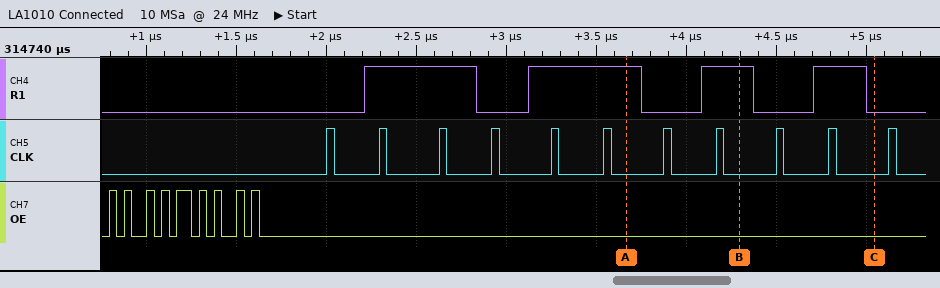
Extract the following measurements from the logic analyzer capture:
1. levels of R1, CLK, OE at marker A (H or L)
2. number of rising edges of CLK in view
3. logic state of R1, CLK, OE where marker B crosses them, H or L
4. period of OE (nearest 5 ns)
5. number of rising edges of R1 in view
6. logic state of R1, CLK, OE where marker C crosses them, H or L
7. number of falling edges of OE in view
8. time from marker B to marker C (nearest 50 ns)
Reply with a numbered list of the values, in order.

1. R1=H, CLK=L, OE=L
2. 11
3. R1=H, CLK=L, OE=L
4. 100 ns
5. 4
6. R1=L, CLK=L, OE=L
7. 9
8. 750 ns
